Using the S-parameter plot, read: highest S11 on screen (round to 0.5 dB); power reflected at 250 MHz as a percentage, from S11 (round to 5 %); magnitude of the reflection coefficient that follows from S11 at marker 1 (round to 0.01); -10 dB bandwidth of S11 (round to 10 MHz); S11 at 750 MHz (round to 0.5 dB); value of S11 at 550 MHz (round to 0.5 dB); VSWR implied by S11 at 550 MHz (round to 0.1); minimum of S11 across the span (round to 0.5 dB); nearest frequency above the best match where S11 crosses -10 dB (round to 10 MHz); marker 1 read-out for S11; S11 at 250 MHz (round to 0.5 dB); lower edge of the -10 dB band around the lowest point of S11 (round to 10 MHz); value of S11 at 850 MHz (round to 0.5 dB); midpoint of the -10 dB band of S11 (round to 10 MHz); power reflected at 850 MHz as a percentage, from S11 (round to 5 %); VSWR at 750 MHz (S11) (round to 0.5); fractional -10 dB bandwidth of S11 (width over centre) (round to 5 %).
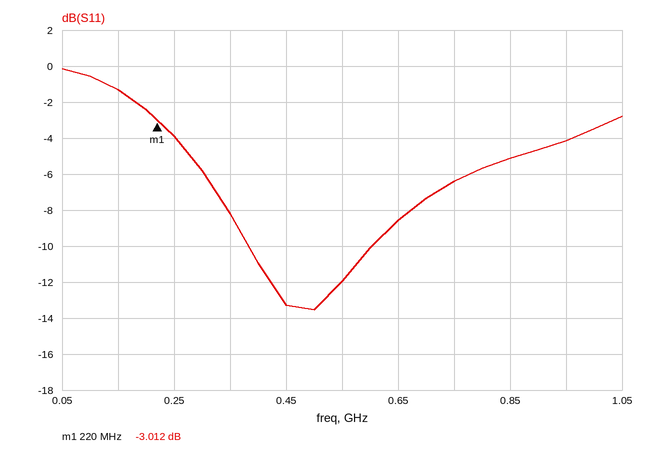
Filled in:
0.0 dB
40 %
0.71
220 MHz
-6.5 dB
-12.0 dB
1.7
-13.5 dB
600 MHz
-3.012 dB
-4.0 dB
380 MHz
-5.0 dB
490 MHz
30 %
3.0
45 %
